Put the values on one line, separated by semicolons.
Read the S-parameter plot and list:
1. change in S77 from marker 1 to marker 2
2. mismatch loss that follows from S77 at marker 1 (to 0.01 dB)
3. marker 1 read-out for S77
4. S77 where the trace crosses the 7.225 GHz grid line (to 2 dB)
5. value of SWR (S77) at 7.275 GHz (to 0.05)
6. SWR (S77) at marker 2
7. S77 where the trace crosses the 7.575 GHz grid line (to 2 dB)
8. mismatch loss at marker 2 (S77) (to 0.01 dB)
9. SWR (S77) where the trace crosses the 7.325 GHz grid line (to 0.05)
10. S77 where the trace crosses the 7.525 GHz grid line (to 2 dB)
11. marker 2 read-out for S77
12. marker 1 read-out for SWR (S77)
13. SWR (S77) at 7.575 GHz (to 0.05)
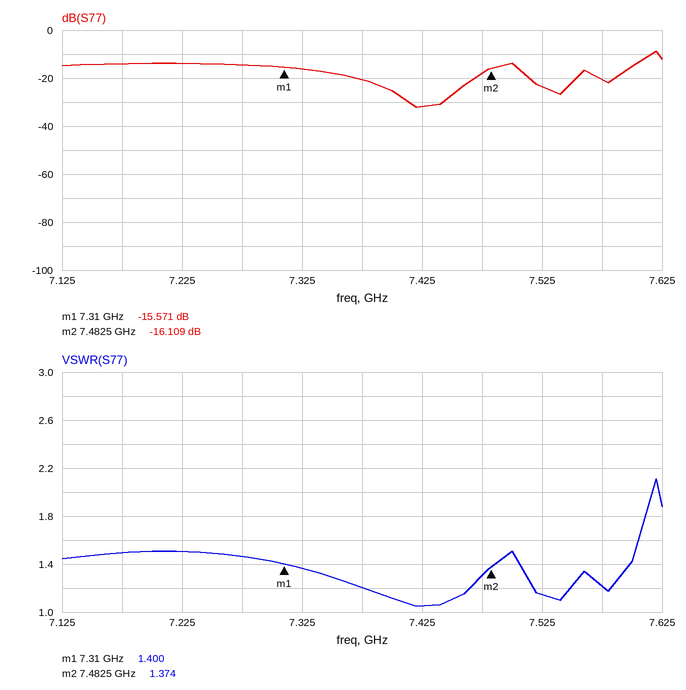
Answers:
-0.538 dB; 0.12 dB; -15.571 dB; -14 dB; 1.45; 1.374; -20 dB; 0.11 dB; 1.35; -24 dB; -16.109 dB; 1.400; 1.20
